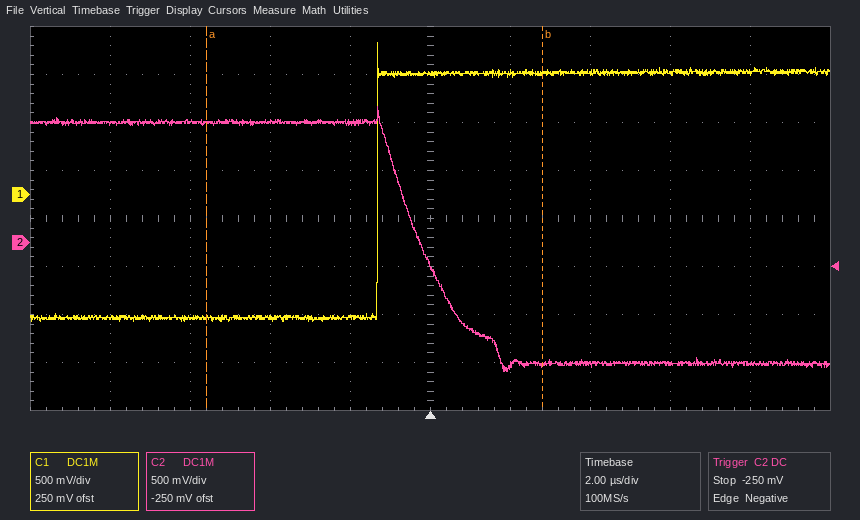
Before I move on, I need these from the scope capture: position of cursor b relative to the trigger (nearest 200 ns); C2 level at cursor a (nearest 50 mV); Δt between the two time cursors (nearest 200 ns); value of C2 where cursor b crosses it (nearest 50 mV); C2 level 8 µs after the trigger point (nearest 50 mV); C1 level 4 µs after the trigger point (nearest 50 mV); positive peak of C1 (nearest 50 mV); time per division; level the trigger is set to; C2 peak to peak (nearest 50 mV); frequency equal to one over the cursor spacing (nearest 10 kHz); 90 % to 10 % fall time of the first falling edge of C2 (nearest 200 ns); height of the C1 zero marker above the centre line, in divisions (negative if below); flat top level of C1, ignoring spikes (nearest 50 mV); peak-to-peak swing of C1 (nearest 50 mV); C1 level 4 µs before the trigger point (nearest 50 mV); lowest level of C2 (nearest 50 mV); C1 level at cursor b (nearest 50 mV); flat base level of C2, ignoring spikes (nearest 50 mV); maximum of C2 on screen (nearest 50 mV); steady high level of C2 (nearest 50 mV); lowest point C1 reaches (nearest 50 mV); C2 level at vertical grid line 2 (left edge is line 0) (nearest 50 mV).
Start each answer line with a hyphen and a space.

- +2.8 µs
- 1.25 V
- 8.4 µs
- -1.25 V
- -1.25 V
- 1.25 V
- 1.60 V
- 2 µs
- -250 mV
- 2.75 V
- 120 kHz
- 2.6 µs
- +0.5 div
- 1.25 V
- 2.90 V
- -1.30 V
- -1.35 V
- 1.25 V
- -1.25 V
- 1.40 V
- 1.25 V
- -1.30 V
- 1.25 V
